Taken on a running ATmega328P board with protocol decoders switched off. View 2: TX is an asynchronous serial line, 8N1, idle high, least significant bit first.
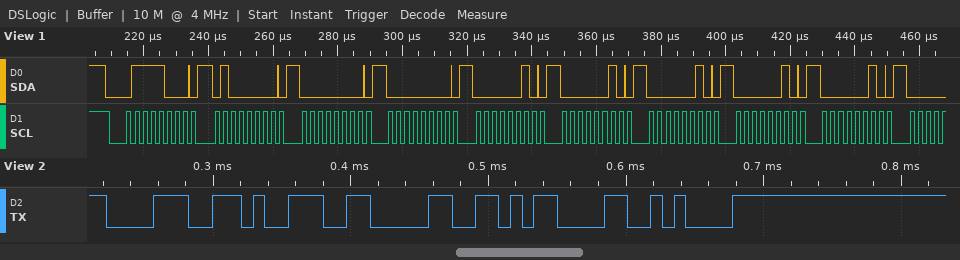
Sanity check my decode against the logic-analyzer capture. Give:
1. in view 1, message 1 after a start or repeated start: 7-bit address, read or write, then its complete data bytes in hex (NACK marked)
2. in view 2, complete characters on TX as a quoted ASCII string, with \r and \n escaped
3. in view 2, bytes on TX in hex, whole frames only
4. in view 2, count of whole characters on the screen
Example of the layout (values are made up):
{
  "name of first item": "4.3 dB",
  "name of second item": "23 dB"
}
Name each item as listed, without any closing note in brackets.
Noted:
{
  "in view 1, message 1 after a start or repeated start: 7-bit address, read or write, then its complete data bytes in hex": "0x3C write: 40 00 00 02 02 02 02 02",
  "in view 2, complete characters on TX as a quoted ASCII string, with \\r and \\n escaped": "\"890\\r\\n\"",
  "in view 2, bytes on TX in hex, whole frames only": "38 39 30 0D 0A",
  "in view 2, count of whole characters on the screen": "5"
}
